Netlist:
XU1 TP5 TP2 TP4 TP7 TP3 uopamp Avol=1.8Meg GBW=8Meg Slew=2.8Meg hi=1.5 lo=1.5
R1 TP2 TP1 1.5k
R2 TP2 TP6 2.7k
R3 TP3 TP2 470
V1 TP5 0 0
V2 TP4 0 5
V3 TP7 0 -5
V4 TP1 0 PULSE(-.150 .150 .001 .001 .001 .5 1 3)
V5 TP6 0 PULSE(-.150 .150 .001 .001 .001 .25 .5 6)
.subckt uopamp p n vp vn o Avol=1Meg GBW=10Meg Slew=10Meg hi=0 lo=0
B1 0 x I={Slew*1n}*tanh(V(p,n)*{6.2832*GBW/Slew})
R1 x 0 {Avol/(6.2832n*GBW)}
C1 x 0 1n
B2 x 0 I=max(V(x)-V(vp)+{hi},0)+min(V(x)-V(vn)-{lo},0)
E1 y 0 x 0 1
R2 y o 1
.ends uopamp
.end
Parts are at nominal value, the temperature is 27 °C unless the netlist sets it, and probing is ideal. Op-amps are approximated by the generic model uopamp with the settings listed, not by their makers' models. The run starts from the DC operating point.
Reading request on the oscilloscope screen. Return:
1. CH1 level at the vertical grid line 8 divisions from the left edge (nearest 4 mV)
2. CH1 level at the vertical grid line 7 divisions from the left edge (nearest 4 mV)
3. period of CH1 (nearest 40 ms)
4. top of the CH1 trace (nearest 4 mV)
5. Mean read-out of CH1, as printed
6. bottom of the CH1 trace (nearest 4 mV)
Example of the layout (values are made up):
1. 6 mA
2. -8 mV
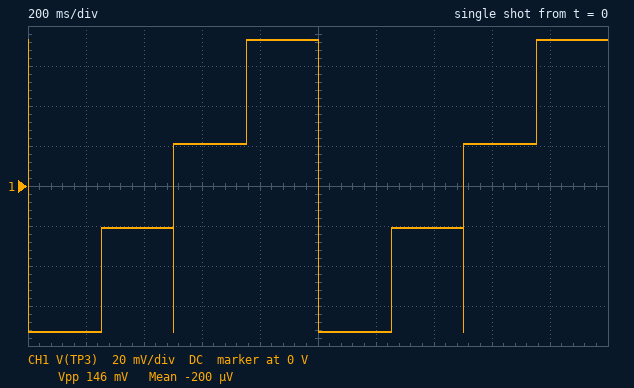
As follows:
1. 20 mV
2. -20 mV
3. 1.00 s
4. 72 mV
5. -200 µV
6. -72 mV
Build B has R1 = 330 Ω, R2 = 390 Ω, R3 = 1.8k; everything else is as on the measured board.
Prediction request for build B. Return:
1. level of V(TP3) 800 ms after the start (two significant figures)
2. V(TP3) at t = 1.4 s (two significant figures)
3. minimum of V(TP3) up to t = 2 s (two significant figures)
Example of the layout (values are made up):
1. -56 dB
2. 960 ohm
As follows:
1. 1.5 V
2. -130 mV
3. -1.5 V
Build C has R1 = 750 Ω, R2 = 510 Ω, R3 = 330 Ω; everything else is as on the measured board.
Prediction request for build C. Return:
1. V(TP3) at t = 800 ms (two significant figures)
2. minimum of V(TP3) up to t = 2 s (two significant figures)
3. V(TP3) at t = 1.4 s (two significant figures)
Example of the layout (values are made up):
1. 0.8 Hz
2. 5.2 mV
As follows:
1. 160 mV
2. -160 mV
3. 31 mV
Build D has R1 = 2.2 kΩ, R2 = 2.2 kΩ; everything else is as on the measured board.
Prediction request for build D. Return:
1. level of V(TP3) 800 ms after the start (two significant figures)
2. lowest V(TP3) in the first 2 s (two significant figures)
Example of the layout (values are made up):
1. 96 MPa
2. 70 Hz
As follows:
1. 64 mV
2. -64 mV
